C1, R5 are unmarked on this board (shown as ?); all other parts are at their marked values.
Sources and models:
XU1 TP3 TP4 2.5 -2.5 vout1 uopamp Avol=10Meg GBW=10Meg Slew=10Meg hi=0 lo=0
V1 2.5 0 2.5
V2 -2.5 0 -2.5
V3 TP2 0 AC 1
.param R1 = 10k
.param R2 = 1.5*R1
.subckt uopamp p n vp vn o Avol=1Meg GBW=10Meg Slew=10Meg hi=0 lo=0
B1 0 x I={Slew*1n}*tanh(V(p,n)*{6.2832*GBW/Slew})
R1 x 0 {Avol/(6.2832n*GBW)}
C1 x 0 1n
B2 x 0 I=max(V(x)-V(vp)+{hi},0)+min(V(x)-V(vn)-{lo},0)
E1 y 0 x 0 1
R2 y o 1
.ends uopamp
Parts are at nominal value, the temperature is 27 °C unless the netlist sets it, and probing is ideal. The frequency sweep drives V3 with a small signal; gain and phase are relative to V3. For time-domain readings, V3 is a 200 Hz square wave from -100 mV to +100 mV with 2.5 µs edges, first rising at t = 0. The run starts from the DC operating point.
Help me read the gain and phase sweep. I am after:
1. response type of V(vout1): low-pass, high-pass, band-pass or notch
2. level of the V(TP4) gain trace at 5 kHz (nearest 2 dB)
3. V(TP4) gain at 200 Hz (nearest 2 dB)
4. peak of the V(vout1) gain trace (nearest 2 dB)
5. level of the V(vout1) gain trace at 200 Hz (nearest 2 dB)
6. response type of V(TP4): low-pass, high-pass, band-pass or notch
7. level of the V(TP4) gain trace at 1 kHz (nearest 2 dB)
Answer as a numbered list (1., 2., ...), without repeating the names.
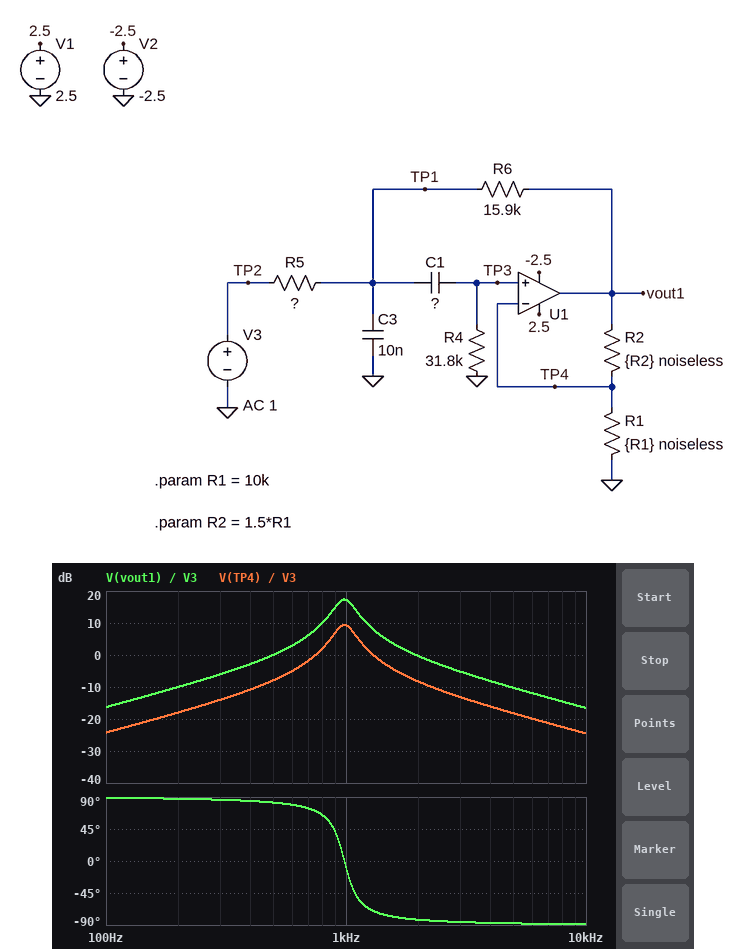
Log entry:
1. band-pass
2. -18 dB
3. -18 dB
4. 18 dB
5. -10 dB
6. band-pass
7. 10 dB
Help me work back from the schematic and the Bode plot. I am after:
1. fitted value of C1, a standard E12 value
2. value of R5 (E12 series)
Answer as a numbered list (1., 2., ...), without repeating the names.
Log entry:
1. 8.2 nF
2. 27 kΩ
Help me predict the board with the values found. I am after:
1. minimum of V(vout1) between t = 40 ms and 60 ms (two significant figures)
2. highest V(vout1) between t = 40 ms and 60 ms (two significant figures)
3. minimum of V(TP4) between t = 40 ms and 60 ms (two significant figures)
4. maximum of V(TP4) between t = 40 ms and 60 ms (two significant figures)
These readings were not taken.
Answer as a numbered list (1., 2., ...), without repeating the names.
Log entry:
1. -320 mV
2. 320 mV
3. -130 mV
4. 130 mV
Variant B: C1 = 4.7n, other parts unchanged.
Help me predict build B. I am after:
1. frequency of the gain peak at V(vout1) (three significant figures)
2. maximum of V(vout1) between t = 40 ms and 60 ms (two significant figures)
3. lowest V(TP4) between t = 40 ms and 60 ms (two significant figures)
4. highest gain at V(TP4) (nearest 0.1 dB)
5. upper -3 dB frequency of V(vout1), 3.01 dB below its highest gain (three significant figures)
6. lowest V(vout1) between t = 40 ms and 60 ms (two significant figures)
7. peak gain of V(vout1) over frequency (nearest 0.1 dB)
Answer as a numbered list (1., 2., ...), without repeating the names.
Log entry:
1. 1.30 kHz
2. 160 mV
3. -64 mV
4. -0.9 dB
5. 1.67 kHz
6. -160 mV
7. 7.1 dB
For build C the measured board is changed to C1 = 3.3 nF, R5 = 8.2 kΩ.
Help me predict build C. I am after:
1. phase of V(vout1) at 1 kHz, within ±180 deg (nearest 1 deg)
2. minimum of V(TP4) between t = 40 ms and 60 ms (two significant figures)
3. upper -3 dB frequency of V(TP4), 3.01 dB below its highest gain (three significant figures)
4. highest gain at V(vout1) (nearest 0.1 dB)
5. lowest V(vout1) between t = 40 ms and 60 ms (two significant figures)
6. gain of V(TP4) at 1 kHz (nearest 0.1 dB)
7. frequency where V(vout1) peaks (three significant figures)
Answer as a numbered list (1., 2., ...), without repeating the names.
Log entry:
1. 55 deg
2. -94 mV
3. 3.67 kHz
4. 5.9 dB
5. -230 mV
6. -6.8 dB
7. 2.11 kHz
